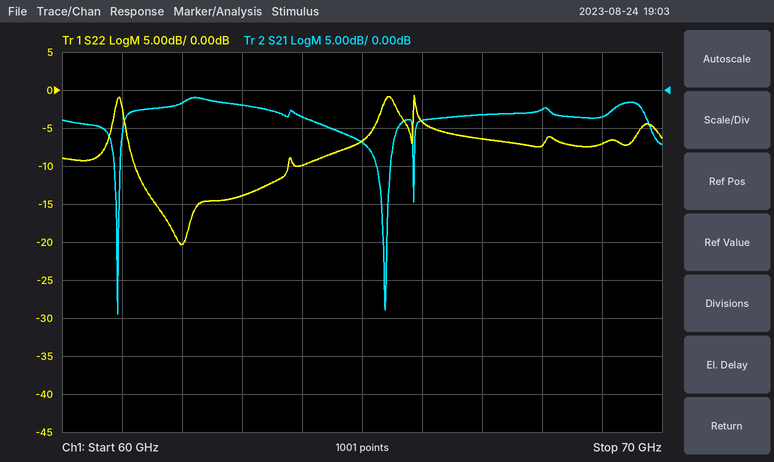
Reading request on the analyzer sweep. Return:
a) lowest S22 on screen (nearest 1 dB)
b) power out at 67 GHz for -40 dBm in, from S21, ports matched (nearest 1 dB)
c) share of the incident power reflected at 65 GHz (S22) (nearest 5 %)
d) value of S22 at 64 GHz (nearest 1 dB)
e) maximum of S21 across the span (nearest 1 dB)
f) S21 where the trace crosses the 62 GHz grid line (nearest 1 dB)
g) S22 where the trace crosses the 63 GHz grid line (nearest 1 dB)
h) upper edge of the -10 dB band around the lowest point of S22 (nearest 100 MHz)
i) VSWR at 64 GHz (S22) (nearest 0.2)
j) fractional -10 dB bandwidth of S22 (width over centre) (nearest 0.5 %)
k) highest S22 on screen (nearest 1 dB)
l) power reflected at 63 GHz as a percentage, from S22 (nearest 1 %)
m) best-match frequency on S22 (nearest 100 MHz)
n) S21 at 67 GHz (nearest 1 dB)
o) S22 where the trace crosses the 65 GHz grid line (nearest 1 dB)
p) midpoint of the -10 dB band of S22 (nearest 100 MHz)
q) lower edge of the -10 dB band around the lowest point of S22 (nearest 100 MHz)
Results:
-20 dB
-43 dBm
20 %
-10 dB
-1 dB
-2 dB
-14 dB
63.8 GHz
2.0
4.0 %
-1 dB
4 %
62.0 GHz
-3 dB
-7 dB
62.5 GHz
61.2 GHz
